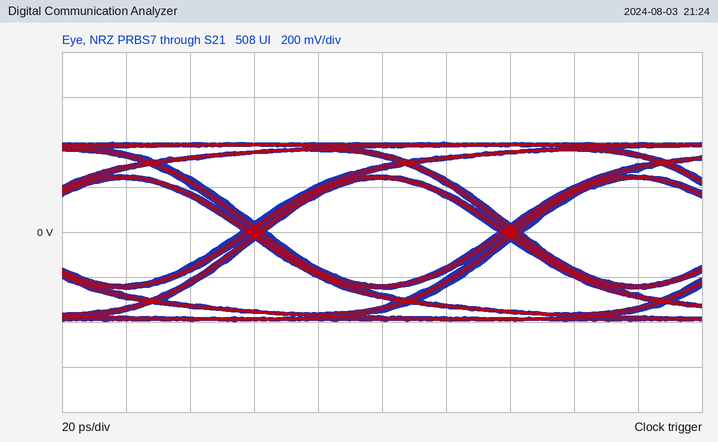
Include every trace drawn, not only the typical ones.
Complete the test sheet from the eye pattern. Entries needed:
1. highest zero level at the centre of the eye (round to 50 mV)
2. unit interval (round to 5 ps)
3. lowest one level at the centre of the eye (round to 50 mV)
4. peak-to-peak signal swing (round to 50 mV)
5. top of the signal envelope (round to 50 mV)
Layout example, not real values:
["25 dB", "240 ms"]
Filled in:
["-250 mV", "80 ps", "250 mV", "800 mV", "400 mV"]
